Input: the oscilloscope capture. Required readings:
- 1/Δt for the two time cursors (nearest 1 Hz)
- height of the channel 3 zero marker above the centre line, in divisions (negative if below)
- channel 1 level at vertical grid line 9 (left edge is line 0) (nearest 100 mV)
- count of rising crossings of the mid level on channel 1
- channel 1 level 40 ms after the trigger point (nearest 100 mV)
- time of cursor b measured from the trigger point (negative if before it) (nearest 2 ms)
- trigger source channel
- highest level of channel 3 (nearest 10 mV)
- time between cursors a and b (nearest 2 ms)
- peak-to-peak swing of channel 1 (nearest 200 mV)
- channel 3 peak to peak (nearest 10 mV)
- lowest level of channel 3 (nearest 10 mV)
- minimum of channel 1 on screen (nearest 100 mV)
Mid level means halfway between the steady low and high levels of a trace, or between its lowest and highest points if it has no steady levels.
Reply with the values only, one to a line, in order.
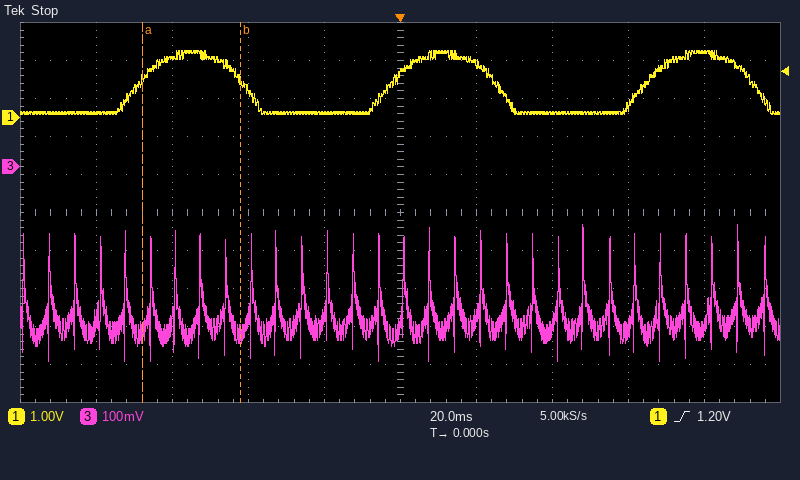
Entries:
38 Hz
+1.2 div
1.7 V
3
100 mV
-42 ms
channel 1
-150 mV
26 ms
1.6 V
360 mV
-510 mV
100 mV
